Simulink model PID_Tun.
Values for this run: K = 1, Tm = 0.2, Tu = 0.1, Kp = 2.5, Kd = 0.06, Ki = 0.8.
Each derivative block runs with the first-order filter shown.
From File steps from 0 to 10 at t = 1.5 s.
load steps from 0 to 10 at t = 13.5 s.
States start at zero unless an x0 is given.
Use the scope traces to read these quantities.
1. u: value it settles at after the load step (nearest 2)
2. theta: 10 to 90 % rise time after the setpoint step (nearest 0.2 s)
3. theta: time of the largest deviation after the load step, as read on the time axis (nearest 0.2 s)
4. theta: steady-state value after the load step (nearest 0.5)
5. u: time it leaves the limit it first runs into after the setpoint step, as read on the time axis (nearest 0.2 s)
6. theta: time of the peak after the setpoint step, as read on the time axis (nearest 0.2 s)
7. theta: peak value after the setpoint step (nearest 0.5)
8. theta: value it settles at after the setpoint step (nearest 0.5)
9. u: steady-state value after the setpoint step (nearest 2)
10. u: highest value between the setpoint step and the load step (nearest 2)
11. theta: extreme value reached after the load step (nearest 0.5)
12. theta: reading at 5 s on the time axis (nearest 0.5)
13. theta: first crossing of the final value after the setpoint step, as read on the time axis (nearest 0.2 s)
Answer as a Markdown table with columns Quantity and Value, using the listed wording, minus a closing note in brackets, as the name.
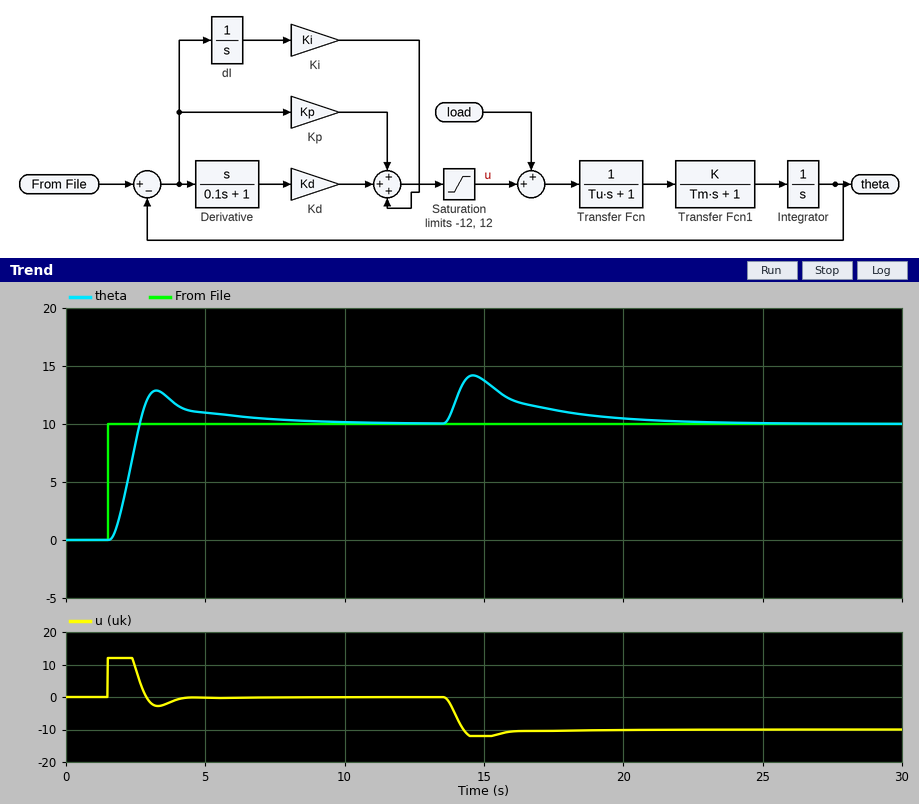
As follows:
| Quantity | Value |
|---|---|
| u: value it settles at after the load step | -10 |
| theta: 10 to 90 % rise time after the setpoint step | 0.8 s |
| theta: time of the largest deviation after the load step, as read on the time axis | 14.6 s |
| theta: steady-state value after the load step | 10.0 |
| u: time it leaves the limit it first runs into after the setpoint step, as read on the time axis | 2.4 s |
| theta: time of the peak after the setpoint step, as read on the time axis | 3.2 s |
| theta: peak value after the setpoint step | 13.0 |
| theta: value it settles at after the setpoint step | 10.0 |
| u: steady-state value after the setpoint step | 0 |
| u: highest value between the setpoint step and the load step | 12 |
| theta: extreme value reached after the load step | 14.0 |
| theta: reading at 5 s on the time axis | 11.0 |
| theta: first crossing of the final value after the setpoint step, as read on the time axis | 2.6 s |
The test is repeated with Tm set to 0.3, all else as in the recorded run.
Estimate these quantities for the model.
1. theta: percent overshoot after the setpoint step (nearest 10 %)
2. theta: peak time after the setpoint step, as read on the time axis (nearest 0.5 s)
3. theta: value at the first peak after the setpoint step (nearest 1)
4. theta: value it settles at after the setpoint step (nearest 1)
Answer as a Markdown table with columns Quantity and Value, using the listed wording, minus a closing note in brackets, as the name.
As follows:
| Quantity | Value |
|---|---|
| theta: percent overshoot after the setpoint step | 40 % |
| theta: peak time after the setpoint step, as read on the time axis | 3.5 s |
| theta: value at the first peak after the setpoint step | 14 |
| theta: value it settles at after the setpoint step | 10 |
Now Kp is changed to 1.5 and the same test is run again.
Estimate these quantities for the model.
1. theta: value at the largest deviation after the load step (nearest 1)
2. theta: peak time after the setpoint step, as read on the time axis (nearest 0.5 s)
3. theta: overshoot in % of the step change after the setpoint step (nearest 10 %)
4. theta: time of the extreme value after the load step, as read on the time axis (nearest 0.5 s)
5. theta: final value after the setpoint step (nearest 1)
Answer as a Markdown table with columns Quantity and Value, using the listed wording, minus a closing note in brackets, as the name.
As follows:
| Quantity | Value |
|---|---|
| theta: value at the largest deviation after the load step | 16 |
| theta: peak time after the setpoint step, as read on the time axis | 3.5 s |
| theta: overshoot in % of the step change after the setpoint step | 30 % |
| theta: time of the extreme value after the load step, as read on the time axis | 15.0 s |
| theta: final value after the setpoint step | 10 |
